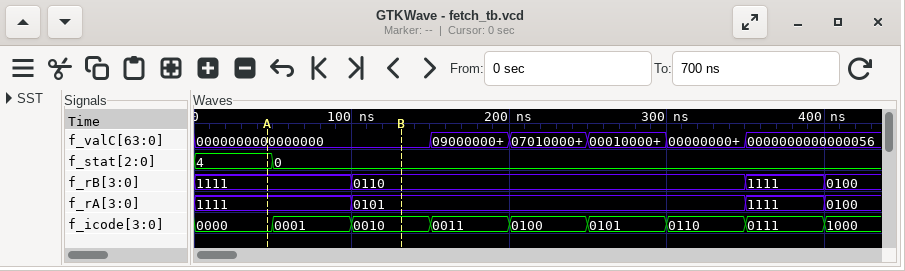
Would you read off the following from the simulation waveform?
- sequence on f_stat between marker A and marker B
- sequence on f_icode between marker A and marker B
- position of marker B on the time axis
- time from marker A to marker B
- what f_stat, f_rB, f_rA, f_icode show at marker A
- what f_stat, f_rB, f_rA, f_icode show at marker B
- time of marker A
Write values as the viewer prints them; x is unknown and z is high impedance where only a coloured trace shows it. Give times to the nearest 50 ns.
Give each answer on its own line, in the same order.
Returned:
4, 0
0000, 0001, 0010
150 ns
100 ns
f_stat=4, f_rB=1111, f_rA=1111, f_icode=0000
f_stat=0, f_rB=0110, f_rA=0101, f_icode=0010
50 ns
